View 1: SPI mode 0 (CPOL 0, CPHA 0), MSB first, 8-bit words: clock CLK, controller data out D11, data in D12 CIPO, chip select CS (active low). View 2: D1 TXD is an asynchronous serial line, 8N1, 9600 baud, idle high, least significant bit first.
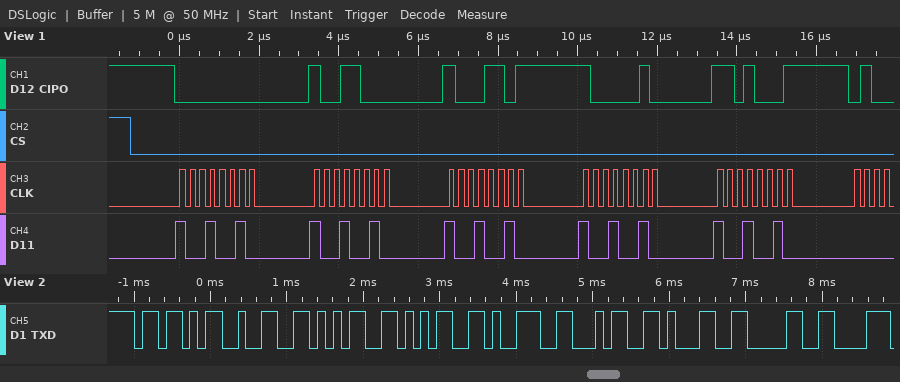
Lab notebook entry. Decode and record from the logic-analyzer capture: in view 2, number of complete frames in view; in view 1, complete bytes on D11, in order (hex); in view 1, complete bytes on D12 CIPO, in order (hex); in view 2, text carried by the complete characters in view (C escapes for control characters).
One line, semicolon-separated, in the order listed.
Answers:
8; 92 92 92 92 92; 00 98 8D 82 D1; "[2559410"
